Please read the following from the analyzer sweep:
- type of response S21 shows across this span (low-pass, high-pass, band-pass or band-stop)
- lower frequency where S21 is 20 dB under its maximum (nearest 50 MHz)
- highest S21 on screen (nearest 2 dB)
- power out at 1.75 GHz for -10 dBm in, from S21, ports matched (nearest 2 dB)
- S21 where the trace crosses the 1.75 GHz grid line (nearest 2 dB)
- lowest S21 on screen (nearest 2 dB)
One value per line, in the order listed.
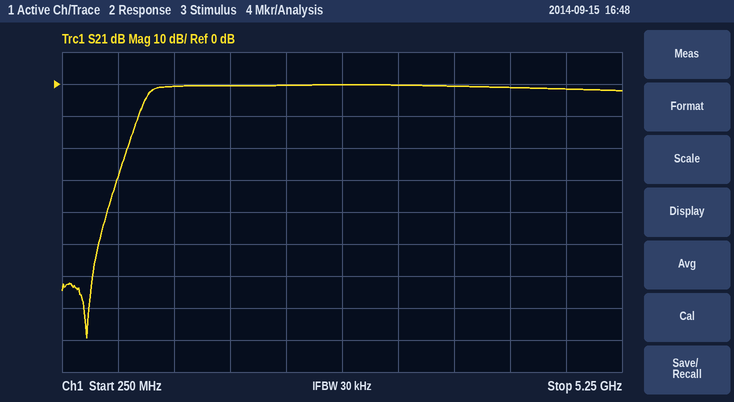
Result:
high-pass
850 MHz
0 dB
-10 dBm
0 dB
-80 dB
